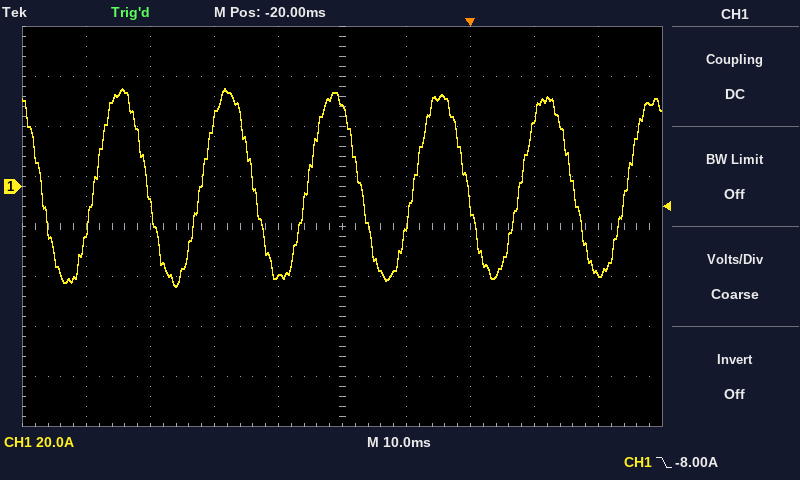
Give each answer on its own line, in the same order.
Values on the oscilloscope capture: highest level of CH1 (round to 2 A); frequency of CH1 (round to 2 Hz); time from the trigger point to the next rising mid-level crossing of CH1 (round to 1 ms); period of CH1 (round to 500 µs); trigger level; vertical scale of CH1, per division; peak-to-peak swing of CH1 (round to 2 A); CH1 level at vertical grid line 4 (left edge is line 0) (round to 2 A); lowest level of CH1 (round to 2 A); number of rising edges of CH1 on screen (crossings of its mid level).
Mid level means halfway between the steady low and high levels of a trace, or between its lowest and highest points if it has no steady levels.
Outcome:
40 A
60 Hz
8 ms
16.5 ms
-8.00 A
20 A
80 A
-36 A
-40 A
6
